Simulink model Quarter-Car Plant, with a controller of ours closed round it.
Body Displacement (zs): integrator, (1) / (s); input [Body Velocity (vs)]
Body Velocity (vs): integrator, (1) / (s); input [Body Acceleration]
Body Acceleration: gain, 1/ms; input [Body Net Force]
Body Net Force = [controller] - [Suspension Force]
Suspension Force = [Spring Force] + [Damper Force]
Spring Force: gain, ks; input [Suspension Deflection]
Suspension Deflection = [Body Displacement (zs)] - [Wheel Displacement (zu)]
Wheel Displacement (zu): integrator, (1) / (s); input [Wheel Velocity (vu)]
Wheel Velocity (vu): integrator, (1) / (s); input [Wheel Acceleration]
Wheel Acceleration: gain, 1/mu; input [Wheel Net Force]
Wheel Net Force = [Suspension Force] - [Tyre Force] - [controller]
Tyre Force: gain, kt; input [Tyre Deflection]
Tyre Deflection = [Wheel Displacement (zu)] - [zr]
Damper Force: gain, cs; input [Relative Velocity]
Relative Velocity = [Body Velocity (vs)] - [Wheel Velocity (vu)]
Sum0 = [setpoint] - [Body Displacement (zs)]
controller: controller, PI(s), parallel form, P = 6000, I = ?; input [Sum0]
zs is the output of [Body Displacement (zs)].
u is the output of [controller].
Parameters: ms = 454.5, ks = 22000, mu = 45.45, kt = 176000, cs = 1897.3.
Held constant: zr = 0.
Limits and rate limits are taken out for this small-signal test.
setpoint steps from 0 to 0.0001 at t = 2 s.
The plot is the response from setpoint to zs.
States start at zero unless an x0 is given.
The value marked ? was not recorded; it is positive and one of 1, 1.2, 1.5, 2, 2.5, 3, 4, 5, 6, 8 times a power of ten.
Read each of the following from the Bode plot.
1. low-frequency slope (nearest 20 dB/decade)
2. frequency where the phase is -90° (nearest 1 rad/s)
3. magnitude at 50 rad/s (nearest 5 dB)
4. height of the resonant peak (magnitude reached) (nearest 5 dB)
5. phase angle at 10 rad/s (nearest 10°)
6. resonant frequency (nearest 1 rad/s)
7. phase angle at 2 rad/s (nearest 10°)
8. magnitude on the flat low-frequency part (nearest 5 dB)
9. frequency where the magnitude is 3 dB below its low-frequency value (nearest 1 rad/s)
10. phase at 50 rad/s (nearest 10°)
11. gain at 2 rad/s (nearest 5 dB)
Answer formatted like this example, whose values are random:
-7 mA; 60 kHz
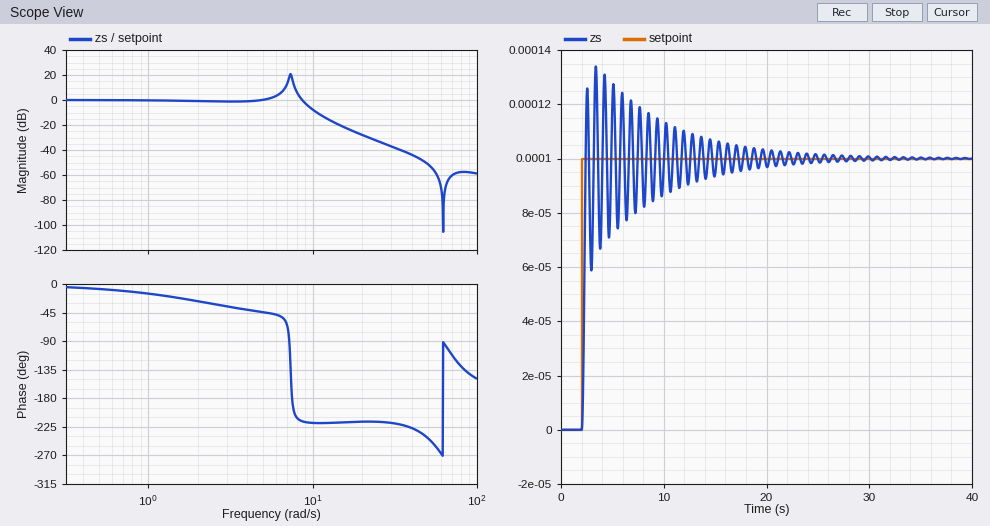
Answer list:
0 dB/decade; 7 rad/s; -50 dB; 20 dB; -220°; 7 rad/s; -30°; 0 dB; 9 rad/s; -240°; 0 dB
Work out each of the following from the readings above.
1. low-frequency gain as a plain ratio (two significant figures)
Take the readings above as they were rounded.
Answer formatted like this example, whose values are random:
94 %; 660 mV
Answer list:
1.0
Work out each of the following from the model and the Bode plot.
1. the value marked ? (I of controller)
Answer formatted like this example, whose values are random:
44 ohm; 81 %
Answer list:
80000
